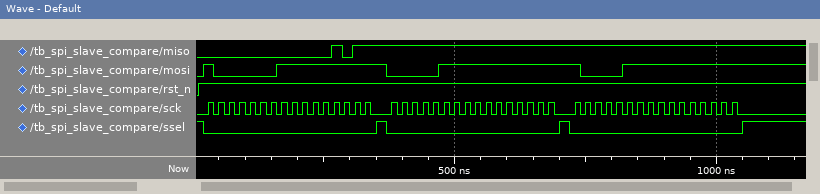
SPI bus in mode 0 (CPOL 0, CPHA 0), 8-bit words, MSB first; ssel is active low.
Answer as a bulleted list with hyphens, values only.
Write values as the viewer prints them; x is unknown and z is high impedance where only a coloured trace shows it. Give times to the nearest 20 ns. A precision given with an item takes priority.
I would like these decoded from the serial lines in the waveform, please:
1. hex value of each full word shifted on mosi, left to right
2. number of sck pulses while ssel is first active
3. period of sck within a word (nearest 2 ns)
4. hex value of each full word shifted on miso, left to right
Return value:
- 81, FF, 07, FF, 87, FF
- 16
- 20 ns
- 00, 0B, FF, FF, FF, FF
